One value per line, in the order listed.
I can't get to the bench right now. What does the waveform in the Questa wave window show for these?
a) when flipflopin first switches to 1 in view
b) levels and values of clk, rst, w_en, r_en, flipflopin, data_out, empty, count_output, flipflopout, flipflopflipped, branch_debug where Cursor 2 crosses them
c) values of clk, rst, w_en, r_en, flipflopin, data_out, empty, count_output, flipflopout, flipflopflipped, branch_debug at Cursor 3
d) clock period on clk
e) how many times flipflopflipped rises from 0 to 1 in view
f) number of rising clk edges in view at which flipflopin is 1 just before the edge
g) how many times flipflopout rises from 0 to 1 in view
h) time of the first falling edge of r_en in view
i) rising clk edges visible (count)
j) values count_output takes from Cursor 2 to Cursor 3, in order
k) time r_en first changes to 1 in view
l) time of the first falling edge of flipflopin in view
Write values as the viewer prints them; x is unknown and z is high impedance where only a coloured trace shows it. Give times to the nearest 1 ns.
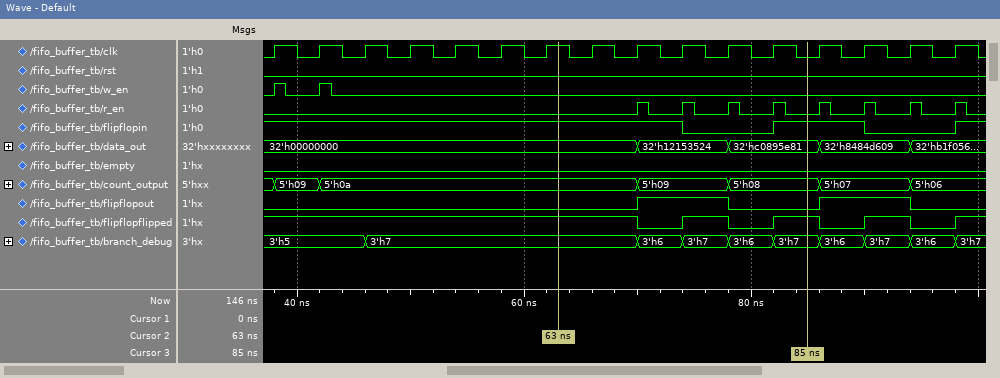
82 ns
clk=1, rst=0, w_en=0, r_en=0, flipflopin=1, data_out=32'h00000000, empty=0, count_output=5'h0a, flipflopout=0, flipflopflipped=1, branch_debug=3'h7
clk=0, rst=0, w_en=0, r_en=0, flipflopin=1, data_out=32'hc0895e81, empty=0, count_output=5'h08, flipflopout=0, flipflopflipped=1, branch_debug=3'h7
4 ns
4
12
2
71 ns
16
5'h0a, 5'h09, 5'h08
70 ns
74 ns
